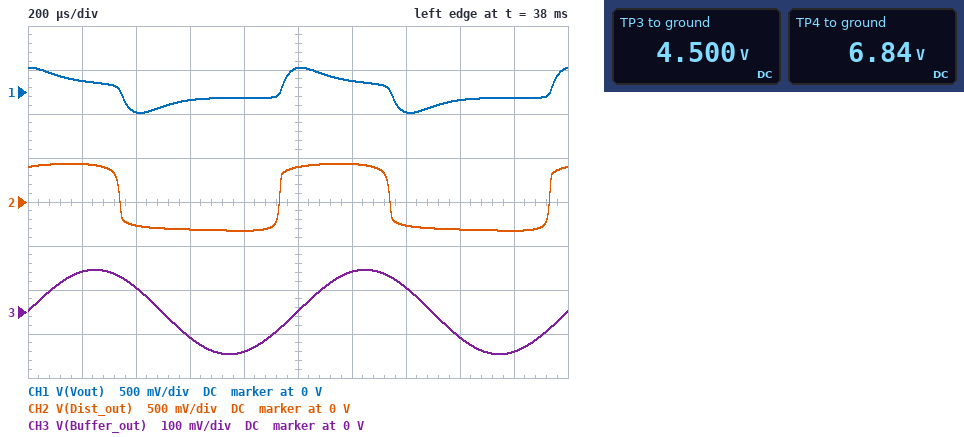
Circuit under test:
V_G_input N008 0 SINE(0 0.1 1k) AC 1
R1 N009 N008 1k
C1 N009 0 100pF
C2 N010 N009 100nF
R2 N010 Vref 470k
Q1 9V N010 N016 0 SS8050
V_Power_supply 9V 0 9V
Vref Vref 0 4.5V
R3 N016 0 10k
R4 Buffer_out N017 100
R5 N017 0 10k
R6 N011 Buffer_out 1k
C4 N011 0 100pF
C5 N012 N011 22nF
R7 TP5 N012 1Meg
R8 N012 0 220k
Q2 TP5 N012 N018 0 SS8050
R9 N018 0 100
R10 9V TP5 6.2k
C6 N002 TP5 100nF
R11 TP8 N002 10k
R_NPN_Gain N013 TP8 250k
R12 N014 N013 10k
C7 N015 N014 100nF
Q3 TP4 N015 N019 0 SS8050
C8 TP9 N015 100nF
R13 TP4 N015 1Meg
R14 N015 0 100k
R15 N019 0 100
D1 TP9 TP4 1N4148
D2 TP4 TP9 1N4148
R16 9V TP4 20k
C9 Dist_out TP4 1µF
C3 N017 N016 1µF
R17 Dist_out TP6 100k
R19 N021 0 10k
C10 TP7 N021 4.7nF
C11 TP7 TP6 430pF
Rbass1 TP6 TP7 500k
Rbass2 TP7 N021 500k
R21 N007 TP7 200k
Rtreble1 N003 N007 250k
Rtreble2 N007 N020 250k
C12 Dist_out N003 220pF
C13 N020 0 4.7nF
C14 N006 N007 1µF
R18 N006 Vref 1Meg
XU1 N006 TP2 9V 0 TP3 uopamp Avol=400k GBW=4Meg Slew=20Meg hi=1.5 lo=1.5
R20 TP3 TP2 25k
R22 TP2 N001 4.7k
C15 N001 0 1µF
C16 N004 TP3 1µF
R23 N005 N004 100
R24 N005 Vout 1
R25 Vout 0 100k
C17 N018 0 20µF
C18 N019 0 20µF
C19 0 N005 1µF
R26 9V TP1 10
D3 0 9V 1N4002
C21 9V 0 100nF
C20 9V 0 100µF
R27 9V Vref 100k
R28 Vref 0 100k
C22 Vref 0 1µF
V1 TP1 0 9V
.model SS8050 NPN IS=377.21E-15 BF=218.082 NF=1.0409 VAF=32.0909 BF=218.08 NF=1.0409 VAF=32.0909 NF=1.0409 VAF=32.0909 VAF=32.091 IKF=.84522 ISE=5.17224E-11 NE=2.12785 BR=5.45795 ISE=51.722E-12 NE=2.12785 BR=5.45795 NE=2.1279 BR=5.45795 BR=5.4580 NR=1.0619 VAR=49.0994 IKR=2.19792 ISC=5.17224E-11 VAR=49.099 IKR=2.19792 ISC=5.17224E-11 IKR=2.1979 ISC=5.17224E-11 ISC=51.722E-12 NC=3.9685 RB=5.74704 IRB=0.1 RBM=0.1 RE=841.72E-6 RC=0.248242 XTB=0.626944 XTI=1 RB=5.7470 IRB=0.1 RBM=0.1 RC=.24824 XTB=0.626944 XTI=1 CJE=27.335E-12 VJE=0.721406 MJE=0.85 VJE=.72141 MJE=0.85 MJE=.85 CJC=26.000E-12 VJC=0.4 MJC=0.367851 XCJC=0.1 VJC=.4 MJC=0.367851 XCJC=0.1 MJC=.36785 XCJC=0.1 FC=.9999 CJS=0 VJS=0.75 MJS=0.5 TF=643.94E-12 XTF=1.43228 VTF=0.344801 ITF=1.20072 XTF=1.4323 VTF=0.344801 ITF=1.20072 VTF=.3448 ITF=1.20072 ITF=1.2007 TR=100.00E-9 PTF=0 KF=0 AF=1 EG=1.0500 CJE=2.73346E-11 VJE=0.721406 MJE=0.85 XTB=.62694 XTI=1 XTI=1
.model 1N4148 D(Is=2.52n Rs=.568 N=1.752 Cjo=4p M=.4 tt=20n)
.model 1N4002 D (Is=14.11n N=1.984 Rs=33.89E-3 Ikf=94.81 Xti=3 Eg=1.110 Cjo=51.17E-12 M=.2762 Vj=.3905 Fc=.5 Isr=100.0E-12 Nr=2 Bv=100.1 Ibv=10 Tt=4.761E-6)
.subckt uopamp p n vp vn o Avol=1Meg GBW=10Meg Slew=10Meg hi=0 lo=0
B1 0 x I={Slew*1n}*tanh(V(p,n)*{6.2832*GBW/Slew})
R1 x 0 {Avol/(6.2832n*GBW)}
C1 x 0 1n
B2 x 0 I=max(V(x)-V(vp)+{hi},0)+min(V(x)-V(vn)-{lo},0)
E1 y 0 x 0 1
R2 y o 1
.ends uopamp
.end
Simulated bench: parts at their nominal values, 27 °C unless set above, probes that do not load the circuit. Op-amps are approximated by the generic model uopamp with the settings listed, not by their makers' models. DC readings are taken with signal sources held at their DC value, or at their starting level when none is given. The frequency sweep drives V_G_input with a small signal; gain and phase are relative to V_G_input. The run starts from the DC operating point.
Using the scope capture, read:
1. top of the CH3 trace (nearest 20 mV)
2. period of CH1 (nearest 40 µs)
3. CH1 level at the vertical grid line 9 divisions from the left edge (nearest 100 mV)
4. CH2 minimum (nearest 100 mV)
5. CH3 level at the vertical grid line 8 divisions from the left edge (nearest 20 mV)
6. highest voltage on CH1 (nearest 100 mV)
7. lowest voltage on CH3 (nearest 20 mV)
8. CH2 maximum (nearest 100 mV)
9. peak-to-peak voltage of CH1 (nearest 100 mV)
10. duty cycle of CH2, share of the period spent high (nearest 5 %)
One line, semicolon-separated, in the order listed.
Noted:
100 mV; 1.00 ms; -100 mV; -300 mV; -60 mV; 300 mV; -100 mV; 400 mV; 500 mV; 40 %
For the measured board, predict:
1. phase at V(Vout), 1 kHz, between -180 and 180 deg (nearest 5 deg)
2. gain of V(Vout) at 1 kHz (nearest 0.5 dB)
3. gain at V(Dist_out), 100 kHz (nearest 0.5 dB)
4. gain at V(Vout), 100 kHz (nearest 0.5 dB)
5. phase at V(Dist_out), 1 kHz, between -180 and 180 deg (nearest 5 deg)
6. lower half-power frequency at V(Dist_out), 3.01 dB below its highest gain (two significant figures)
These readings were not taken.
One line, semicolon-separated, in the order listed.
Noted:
70 deg; 32.0 dB; 25.0 dB; -5.0 dB; 45 deg; 960 Hz
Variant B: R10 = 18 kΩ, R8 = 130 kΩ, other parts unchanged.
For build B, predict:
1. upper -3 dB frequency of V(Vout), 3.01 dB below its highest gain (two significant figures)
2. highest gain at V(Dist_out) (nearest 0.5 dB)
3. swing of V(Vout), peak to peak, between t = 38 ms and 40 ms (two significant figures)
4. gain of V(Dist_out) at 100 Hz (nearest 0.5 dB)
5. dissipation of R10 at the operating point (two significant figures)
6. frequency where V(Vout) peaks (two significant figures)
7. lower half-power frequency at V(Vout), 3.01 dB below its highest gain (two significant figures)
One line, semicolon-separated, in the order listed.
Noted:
6.0 kHz; 43.0 dB; 520 mV; 25.0 dB; 460 µW; 2.7 kHz; 1.3 kHz
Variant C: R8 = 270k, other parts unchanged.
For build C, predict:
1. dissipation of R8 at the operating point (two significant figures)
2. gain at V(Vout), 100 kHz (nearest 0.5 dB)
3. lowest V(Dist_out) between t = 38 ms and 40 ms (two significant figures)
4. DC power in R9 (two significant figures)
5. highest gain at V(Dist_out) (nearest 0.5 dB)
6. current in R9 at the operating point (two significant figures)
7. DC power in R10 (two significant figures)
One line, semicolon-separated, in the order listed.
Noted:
1.4 µW; -4.5 dB; -340 mV; 22 µW; 43.0 dB; 470 µA; 1.4 mW
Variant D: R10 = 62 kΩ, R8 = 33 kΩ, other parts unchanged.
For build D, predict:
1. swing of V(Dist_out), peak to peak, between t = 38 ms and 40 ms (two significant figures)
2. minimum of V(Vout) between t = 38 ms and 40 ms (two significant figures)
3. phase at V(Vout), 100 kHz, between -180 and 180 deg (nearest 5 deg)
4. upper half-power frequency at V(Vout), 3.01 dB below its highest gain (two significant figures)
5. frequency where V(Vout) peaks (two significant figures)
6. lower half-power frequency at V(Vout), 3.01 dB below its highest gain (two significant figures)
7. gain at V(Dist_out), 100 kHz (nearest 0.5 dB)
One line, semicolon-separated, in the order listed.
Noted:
24 mV; -5.9 mV; 60 deg; 6.6 kHz; 2.6 kHz; 1.1 kHz; -23.0 dB
